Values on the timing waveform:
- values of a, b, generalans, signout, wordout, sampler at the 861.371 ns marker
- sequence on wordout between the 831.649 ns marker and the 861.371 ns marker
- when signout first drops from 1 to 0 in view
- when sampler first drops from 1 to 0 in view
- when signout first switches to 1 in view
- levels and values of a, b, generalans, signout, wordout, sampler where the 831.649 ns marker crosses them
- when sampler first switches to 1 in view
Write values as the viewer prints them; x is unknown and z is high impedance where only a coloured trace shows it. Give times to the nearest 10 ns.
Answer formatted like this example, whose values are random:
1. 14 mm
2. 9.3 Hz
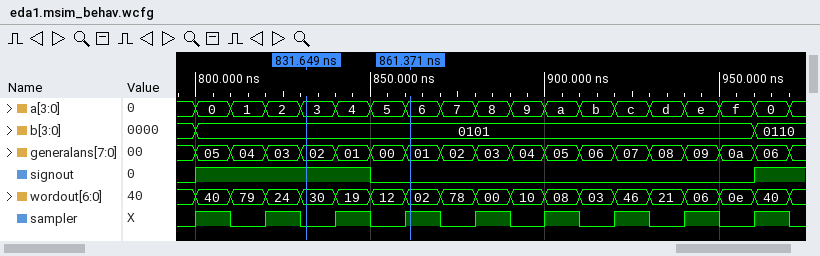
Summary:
1. a=6, b=0101, generalans=01, signout=0, wordout=02, sampler=1
2. 30, 19, 12, 02
3. 850 ns
4. 810 ns
5. 800 ns
6. a=3, b=0101, generalans=02, signout=1, wordout=30, sampler=0
7. 800 ns
